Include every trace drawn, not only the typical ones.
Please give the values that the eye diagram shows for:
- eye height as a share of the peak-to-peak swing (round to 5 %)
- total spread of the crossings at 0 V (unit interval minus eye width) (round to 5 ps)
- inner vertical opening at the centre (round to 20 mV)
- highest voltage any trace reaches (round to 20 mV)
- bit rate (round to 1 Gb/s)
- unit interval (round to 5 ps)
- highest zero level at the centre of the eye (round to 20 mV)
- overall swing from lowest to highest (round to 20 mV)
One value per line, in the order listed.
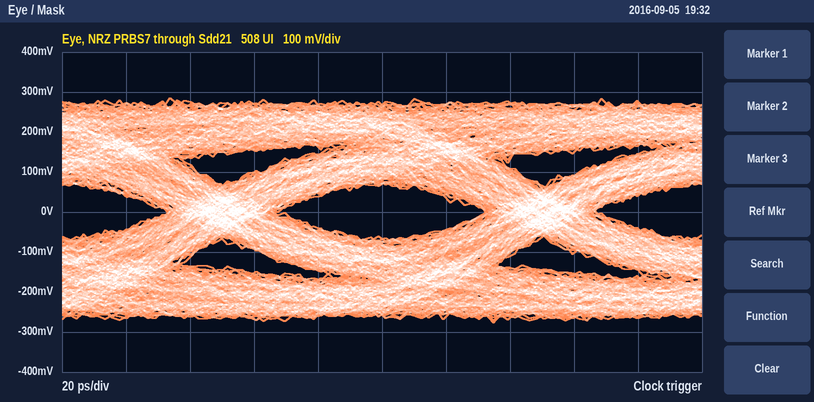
25 %
35 ps
140 mV
280 mV
10 Gb/s
100 ps
-60 mV
560 mV
